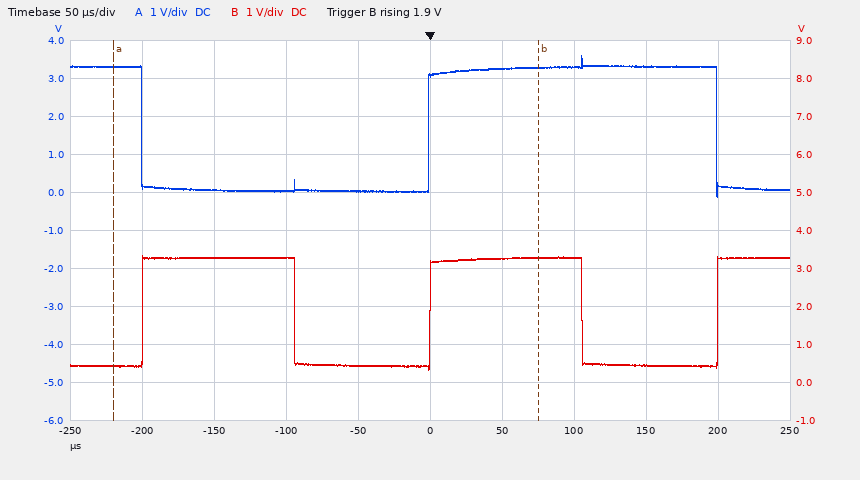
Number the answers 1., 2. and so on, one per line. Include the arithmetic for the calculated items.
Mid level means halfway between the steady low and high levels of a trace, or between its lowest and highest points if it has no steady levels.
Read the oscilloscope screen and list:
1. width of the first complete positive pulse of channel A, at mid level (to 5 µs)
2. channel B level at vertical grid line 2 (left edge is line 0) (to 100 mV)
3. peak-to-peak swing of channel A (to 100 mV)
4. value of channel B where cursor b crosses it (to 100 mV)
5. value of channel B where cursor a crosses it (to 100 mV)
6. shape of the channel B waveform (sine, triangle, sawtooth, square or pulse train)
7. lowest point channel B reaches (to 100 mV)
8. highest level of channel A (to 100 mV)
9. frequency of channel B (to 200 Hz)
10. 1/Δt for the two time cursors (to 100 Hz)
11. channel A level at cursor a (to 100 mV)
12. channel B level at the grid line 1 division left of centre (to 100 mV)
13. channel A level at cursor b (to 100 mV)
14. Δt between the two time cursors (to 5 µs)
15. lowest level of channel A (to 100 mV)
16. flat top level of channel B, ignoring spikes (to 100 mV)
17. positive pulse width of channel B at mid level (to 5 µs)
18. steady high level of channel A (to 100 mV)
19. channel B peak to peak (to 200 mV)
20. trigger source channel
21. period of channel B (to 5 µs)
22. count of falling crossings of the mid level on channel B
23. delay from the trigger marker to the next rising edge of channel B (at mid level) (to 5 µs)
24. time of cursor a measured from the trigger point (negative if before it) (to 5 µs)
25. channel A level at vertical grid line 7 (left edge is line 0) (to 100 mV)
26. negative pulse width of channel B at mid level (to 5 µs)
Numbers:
1. 200 µs
2. 3.3 V
3. 3.6 V − (-100 mV) = 3.7 V
4. 3.3 V
5. 400 mV
6. square
7. 300 mV
8. 3.6 V
9. 1 / 200 µs ≈ 5.0 kHz
10. 1 / 295 µs ≈ 3.4 kHz
11. 3.3 V
12. 400 mV
13. 3.3 V
14. 295 µs
15. -100 mV
16. 3.3 V
17. 105 µs
18. 3.3 V
19. 3.0 V
20. channel B
21. 200 µs
22. 2
23. 200 µs
24. -220 µs
25. 3.3 V
26. 95 µs
